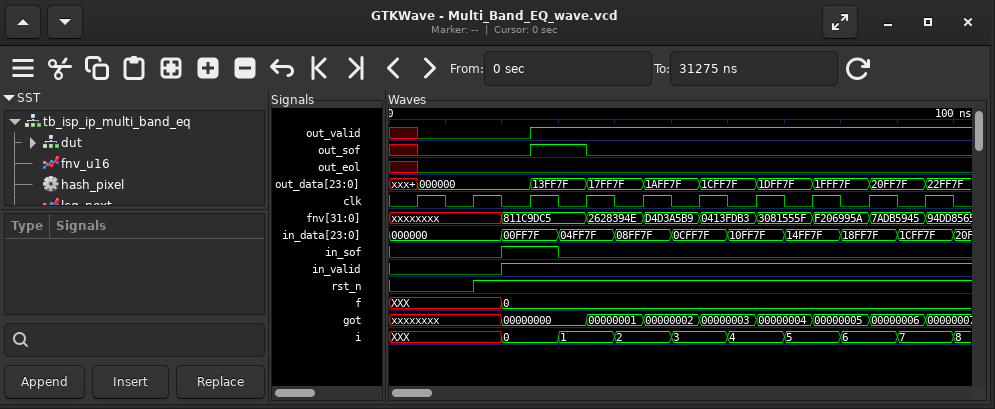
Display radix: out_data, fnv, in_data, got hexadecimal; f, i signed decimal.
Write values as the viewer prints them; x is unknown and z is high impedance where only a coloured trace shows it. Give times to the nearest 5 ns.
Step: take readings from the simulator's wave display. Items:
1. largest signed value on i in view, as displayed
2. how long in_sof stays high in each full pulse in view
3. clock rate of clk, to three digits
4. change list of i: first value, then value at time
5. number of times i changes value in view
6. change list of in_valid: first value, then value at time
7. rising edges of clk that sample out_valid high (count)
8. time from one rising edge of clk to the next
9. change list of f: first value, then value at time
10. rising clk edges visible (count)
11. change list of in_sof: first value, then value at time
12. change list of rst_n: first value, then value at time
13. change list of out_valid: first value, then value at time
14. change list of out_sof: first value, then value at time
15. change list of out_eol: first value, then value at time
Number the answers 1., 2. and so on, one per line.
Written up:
1. 8
2. 10 ns
3. 100 MHz
4. XXX, 0 at 20 ns, 1 at 30 ns, 2 at 40 ns, 3 at 50 ns, 4 at 60 ns, 5 at 70 ns, 6 at 80 ns, 7 at 90 ns, 8 at 100 ns
5. 9
6. 0, 1 at 20 ns
7. 7
8. 10 ns
9. XXX, 0 at 20 ns
10. 10
11. 0, 1 at 20 ns, 0 at 30 ns
12. 0, 1 at 15 ns
13. x, 0 at 5 ns, 1 at 25 ns
14. x, 0 at 5 ns, 1 at 25 ns, 0 at 35 ns
15. x, 0 at 5 ns
